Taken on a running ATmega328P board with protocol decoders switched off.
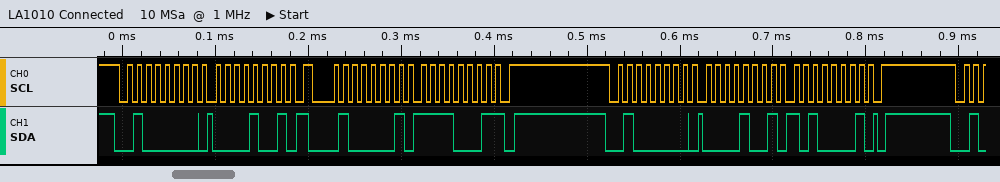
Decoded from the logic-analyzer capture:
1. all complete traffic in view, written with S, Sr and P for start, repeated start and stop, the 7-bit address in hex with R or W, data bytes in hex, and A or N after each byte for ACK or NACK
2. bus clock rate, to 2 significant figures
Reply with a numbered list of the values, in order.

1. S 20W A 09 A Sr 20R A F1 N P S 20W A 09 A A1 A P
2. 100 kHz
